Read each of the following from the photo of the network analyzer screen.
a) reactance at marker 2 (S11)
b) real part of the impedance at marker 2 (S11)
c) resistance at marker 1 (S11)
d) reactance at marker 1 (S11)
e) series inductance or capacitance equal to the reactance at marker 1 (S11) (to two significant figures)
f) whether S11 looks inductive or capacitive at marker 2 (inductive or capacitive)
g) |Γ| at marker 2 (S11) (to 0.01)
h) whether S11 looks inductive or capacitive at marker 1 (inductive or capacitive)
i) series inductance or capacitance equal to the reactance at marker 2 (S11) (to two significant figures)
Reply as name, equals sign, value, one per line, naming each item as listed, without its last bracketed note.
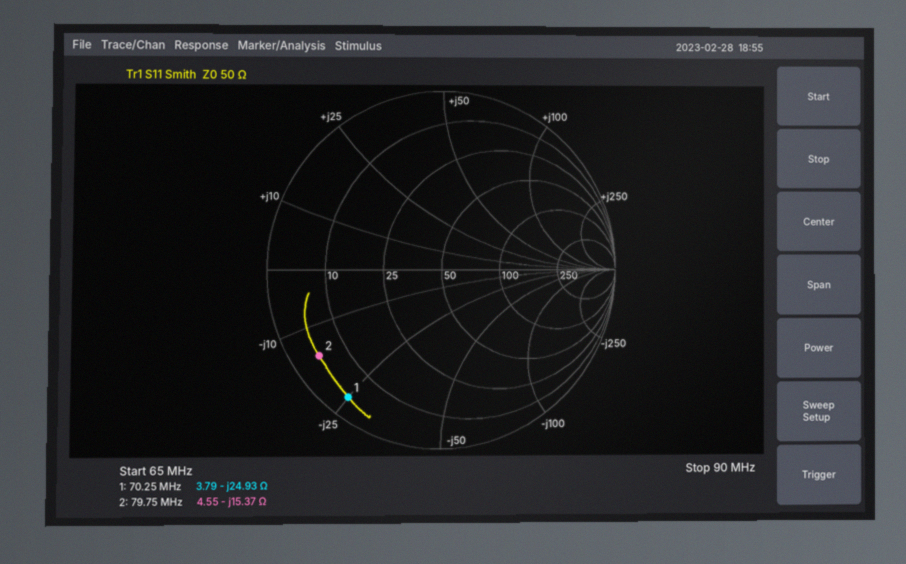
reactance at marker 2 = -15.37 Ω
real part of the impedance at marker 2 = 4.55 Ω
resistance at marker 1 = 3.79 Ω
reactance at marker 1 = -24.93 Ω
series inductance or capacitance equal to the reactance at marker 1 (S11) = 91 pF
whether S11 looks inductive or capacitive at marker 2 = capacitive
|Γ| at marker 2 (S11) = 0.85
whether S11 looks inductive or capacitive at marker 1 = capacitive
series inductance or capacitance equal to the reactance at marker 2 (S11) = 130 pF
